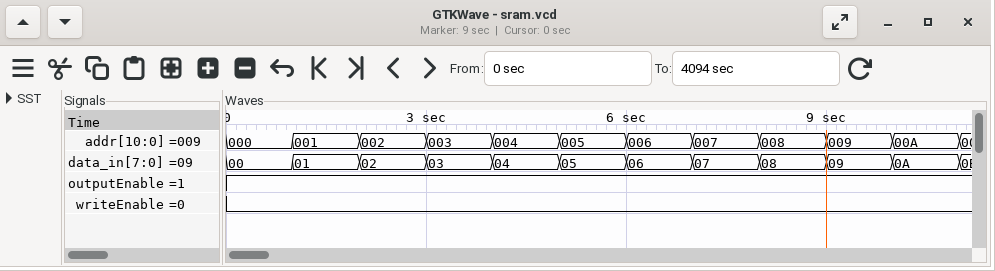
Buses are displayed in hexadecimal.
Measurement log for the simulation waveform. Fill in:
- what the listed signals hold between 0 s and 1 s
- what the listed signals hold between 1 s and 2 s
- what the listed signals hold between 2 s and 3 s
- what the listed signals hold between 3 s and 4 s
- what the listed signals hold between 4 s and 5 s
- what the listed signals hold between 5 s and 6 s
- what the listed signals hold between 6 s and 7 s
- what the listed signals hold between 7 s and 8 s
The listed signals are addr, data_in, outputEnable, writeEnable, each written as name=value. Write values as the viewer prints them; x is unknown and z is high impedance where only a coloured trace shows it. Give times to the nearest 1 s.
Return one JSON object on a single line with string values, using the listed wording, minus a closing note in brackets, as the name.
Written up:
{"what the listed signals hold between 0 s and 1 s": "addr=000, data_in=00, outputEnable=1, writeEnable=0", "what the listed signals hold between 1 s and 2 s": "addr=001, data_in=01, outputEnable=1, writeEnable=0", "what the listed signals hold between 2 s and 3 s": "addr=002, data_in=02, outputEnable=1, writeEnable=0", "what the listed signals hold between 3 s and 4 s": "addr=003, data_in=03, outputEnable=1, writeEnable=0", "what the listed signals hold between 4 s and 5 s": "addr=004, data_in=04, outputEnable=1, writeEnable=0", "what the listed signals hold between 5 s and 6 s": "addr=005, data_in=05, outputEnable=1, writeEnable=0", "what the listed signals hold between 6 s and 7 s": "addr=006, data_in=06, outputEnable=1, writeEnable=0", "what the listed signals hold between 7 s and 8 s": "addr=007, data_in=07, outputEnable=1, writeEnable=0"}
